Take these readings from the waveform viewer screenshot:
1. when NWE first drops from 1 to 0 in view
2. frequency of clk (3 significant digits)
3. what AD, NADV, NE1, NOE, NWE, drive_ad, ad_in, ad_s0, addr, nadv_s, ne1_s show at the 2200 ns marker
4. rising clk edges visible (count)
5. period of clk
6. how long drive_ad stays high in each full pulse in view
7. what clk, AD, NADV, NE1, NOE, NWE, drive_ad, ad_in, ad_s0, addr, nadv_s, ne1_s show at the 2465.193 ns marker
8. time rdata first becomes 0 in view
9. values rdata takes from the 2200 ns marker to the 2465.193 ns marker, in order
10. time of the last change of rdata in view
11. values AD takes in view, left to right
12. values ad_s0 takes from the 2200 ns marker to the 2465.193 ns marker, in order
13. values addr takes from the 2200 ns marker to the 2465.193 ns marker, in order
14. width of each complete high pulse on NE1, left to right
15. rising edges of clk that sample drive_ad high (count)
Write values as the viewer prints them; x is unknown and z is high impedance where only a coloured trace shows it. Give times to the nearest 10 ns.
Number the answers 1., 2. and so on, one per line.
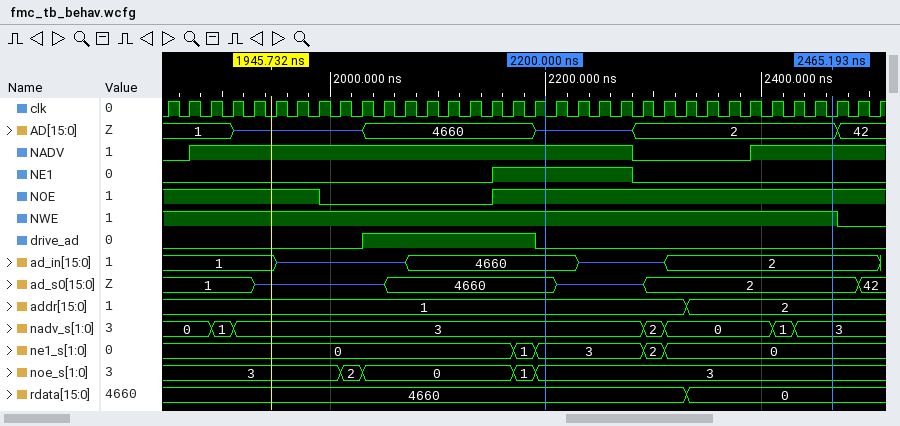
1. 2470 ns
2. 50.0 MHz
3. AD=z, NADV=1, NE1=1, NOE=1, NWE=1, drive_ad=0, ad_in=4660, ad_s0=4660, addr=1, nadv_s=3, ne1_s=3
4. 34
5. 20 ns
6. 160 ns
7. clk=0, AD=2, NADV=1, NE1=0, NOE=1, NWE=1, drive_ad=0, ad_in=2, ad_s0=2, addr=2, nadv_s=3, ne1_s=0
8. 2330 ns
9. 4660, 0
10. 2330 ns
11. 1, z, 4660, z, 2, 42
12. 4660, z, 2
13. 1, 2
14. 130 ns
15. 8
